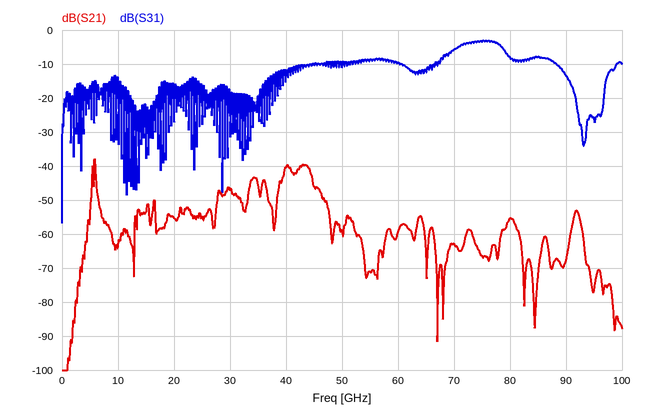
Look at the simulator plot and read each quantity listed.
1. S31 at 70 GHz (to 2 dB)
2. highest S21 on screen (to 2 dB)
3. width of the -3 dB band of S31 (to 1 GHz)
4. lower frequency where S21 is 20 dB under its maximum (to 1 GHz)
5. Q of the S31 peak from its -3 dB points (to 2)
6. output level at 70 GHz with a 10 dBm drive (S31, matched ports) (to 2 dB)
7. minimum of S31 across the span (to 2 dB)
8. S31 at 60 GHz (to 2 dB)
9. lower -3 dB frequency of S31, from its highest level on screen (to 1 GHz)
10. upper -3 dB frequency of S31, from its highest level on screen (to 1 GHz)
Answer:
-6 dB
-38 dB
9 GHz
5 GHz
8
4 dBm
-56 dB
-10 dB
70 GHz
79 GHz
